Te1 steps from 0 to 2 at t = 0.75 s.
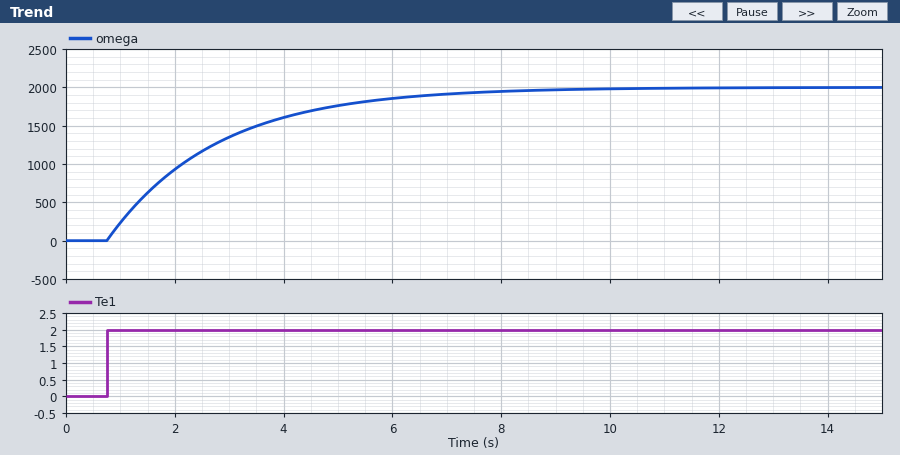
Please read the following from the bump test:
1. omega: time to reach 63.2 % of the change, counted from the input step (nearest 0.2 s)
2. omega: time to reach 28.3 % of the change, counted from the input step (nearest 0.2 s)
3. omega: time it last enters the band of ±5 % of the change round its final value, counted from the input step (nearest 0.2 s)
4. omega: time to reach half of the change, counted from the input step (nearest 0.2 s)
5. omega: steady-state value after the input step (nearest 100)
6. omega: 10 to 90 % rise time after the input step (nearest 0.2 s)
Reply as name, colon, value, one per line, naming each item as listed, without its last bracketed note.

omega: time to reach 63.2 % of the change, counted from the input step: 2.0 s
omega: time to reach 28.3 % of the change, counted from the input step: 0.6 s
omega: time it last enters the band of ±5 % of the change round its final value, counted from the input step: 6.0 s
omega: time to reach half of the change, counted from the input step: 1.4 s
omega: steady-state value after the input step: 2000
omega: 10 to 90 % rise time after the input step: 4.4 s
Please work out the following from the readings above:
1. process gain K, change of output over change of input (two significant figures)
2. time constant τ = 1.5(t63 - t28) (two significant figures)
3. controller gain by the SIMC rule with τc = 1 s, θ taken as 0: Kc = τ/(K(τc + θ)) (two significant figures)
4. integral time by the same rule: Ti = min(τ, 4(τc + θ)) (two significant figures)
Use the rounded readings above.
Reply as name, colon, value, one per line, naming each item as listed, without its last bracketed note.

process gain K, change of output over change of input: 1000
time constant τ = 1.5(t63 - t28): 2.1 s
controller gain by the SIMC rule with τc = 1 s, θ taken as 0: Kc = τ/(K(τc + θ)): 0.0021
integral time by the same rule: Ti = min(τ, 4(τc + θ)): 2.1 s
